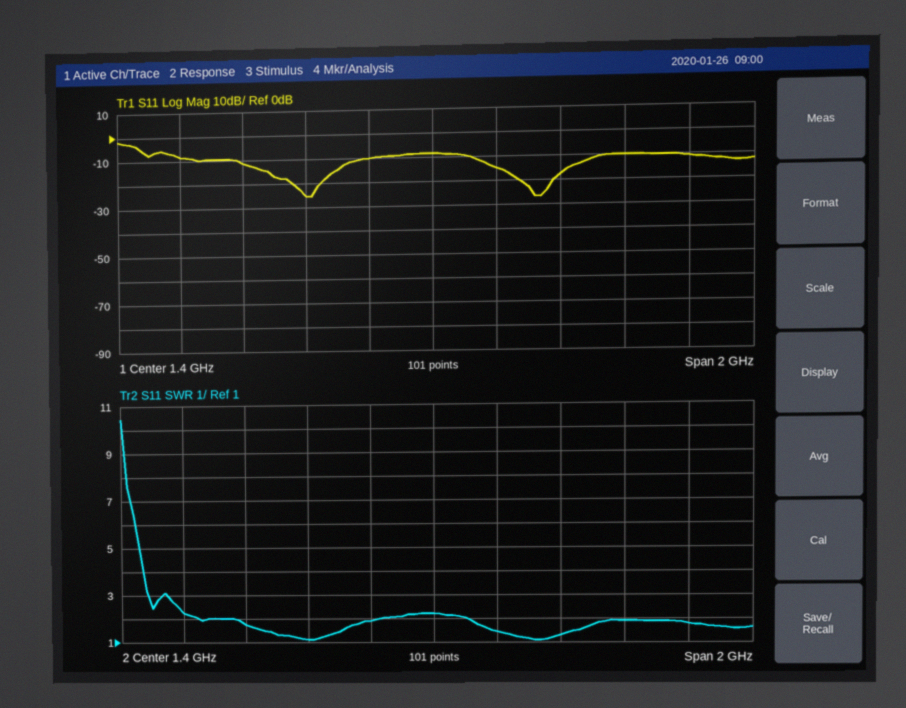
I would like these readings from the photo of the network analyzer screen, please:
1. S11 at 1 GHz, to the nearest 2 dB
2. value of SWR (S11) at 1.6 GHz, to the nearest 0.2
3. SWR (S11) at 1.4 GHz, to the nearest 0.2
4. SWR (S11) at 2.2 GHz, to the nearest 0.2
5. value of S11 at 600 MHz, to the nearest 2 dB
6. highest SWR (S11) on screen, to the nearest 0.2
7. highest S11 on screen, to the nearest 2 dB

-26 dB
1.4
2.2
1.8
-8 dB
10.4
-2 dB
